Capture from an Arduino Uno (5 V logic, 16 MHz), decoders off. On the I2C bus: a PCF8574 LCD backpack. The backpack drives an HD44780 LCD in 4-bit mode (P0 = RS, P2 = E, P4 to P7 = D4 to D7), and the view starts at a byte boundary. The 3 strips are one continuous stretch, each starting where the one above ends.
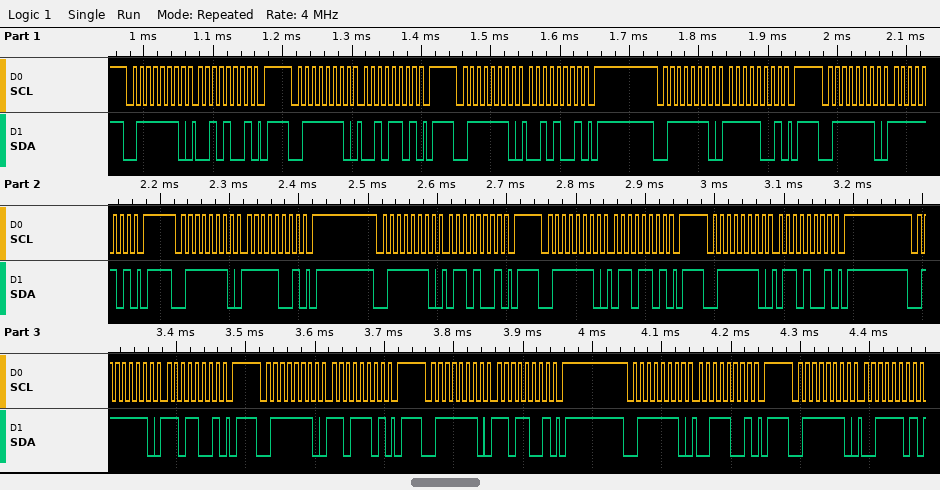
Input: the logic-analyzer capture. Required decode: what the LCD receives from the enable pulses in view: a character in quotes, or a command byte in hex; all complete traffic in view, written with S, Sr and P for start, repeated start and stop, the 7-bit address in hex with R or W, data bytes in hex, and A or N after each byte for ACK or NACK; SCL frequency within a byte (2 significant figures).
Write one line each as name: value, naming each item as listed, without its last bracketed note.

what the LCD receives from the enable pulses in view: a character in quotes, or a command byte in hex: '/' 'm'
all complete traffic in view, written with S, Sr and P for start, repeated start and stop, the 7-bit address in hex with R or W, data bytes in hex, and A or N after each byte for ACK or NACK: S 3FW A 29 A P S 3FW A 2D A P S 3FW A 29 A P S 3FW A F9 A P S 3FW A FD A P S 3FW A F9 A P S 3FW A 69 A P S 3FW A 6D A P S 3FW A 69 A P S 3FW A D9 A P S 3FW A DD A P S 3FW A D9 A P S 3FW A 39 A P S 3FW A 3D A
SCL frequency within a byte: 100 kHz
